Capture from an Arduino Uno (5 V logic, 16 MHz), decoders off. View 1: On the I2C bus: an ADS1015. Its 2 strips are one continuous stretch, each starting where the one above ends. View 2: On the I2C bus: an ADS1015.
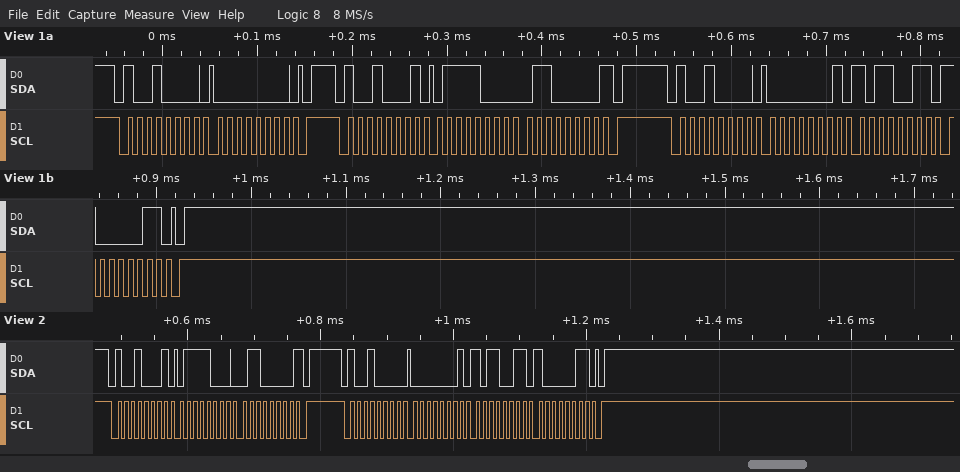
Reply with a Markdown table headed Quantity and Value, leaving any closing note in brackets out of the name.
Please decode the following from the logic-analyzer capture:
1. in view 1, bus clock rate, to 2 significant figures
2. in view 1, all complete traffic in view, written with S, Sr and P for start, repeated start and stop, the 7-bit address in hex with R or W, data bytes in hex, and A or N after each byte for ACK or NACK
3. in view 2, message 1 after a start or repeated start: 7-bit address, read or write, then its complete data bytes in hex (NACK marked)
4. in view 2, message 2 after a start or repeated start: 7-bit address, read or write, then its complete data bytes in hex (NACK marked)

| Quantity | Value |
|---|---|
| in view 1, bus clock rate, to 2 significant figures | 100 kHz |
| in view 1, all complete traffic in view, written with S, Sr and P for start, repeated start and stop, the 7-bit address in hex with R or W, data bytes in hex, and A or N after each byte for ACK or NACK | S 48W A 00 A P S 48R A 78 A 60 N P S 48W A 01 A B3 A 83 A P |
| in view 2, message 1 after a start or repeated start: 7-bit address, read or write, then its complete data bytes in hex | 0x48 read: 78 60 NACK |
| in view 2, message 2 after a start or repeated start: 7-bit address, read or write, then its complete data bytes in hex | 0x48 write: 01 B3 83 |
